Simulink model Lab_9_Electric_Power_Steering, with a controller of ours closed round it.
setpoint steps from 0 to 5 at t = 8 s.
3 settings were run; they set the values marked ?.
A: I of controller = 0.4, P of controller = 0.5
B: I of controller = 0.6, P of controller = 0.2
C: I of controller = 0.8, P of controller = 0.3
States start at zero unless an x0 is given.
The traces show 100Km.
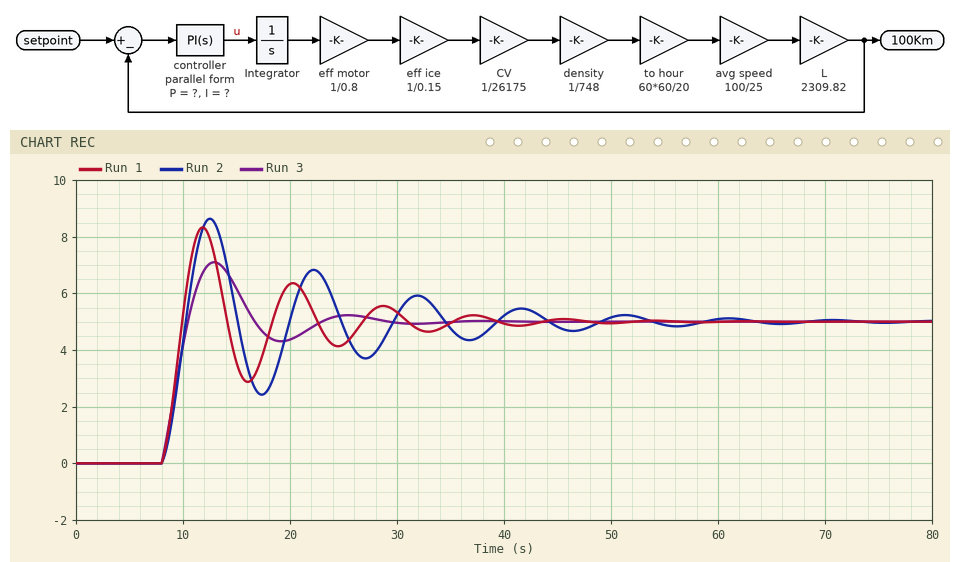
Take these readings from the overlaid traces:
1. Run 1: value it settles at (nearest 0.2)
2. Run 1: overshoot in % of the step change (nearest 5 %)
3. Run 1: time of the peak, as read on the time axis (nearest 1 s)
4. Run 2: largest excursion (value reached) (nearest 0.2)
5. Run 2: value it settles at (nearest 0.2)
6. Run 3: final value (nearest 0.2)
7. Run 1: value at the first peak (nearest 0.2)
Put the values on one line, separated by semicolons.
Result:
5.0; 65 %; 12 s; 8.6; 5.0; 5.0; 8.4
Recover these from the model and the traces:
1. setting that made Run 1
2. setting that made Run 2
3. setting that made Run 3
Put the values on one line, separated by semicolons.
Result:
C; B; A
